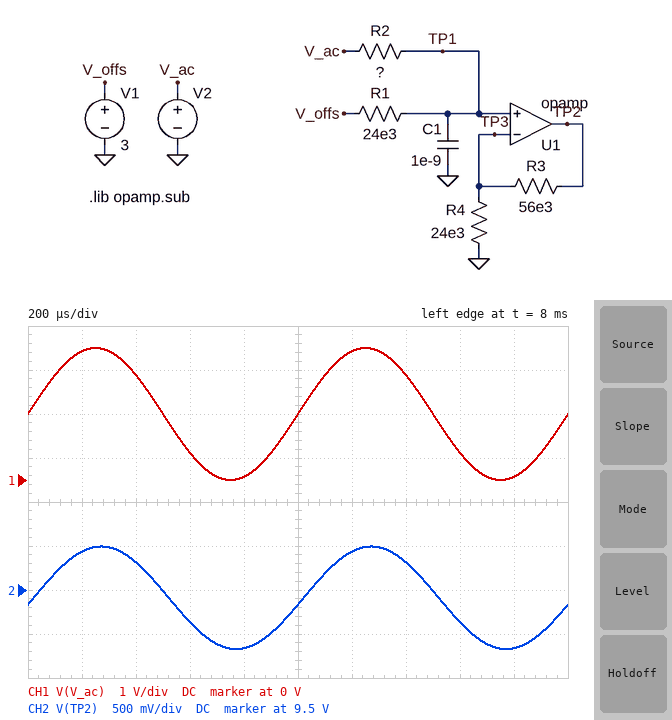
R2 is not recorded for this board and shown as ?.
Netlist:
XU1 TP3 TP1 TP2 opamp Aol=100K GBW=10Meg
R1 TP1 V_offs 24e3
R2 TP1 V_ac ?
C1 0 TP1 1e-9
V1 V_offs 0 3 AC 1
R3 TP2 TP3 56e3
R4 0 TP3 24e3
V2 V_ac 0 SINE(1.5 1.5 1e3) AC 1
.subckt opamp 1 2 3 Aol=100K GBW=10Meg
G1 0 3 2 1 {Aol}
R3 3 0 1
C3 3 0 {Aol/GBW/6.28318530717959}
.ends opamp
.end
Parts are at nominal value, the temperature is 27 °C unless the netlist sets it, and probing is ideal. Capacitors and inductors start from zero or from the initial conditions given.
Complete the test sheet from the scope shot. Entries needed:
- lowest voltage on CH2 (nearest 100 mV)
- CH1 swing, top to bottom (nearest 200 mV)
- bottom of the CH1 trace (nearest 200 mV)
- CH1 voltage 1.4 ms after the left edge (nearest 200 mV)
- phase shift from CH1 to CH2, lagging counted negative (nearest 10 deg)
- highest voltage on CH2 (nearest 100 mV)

8.8 V
3.0 V
0 V
2.4 V
-10 deg
10.0 V
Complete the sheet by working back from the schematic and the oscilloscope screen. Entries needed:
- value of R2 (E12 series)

180 kΩ
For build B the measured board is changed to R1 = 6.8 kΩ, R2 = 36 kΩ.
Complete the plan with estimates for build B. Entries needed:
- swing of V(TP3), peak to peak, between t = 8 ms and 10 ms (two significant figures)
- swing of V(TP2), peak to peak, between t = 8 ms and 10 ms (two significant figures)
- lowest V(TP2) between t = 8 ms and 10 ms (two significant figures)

480 mV
1.6 V
8.4 V
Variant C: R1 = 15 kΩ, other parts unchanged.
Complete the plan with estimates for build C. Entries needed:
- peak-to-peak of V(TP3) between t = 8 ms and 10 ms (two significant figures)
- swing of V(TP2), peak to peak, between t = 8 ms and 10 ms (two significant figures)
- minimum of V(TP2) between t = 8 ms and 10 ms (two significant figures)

230 mV
770 mV
9.2 V
